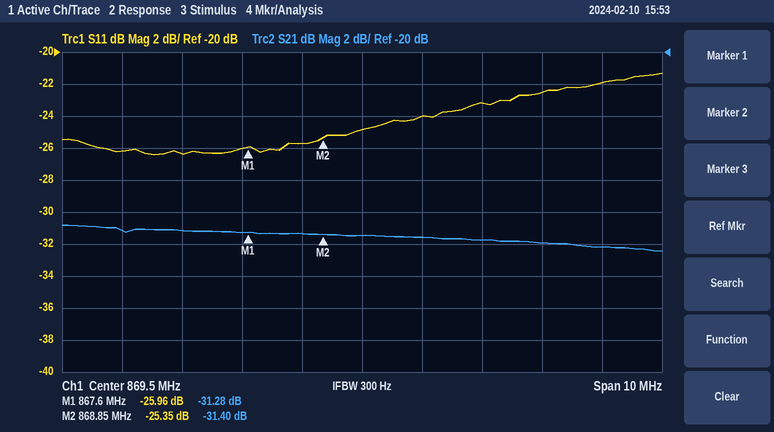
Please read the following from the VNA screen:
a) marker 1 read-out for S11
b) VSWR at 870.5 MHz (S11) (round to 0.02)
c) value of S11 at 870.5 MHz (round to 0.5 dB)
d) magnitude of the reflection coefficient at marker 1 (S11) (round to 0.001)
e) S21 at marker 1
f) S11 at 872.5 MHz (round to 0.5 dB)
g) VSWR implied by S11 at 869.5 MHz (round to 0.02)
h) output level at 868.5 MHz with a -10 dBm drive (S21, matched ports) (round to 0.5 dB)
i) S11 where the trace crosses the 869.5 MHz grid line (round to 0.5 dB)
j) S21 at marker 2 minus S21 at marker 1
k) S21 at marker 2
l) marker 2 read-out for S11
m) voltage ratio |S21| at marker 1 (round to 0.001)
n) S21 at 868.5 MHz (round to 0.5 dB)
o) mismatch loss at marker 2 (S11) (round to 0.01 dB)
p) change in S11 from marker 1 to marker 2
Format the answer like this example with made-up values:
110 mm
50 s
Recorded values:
-25.96 dB
1.14
-24.0 dB
0.050
-31.28 dB
-22.5 dB
1.12
-41.5 dBm
-25.0 dB
-0.12 dB
-31.40 dB
-25.35 dB
0.027
-31.5 dB
0.01 dB
0.61 dB
